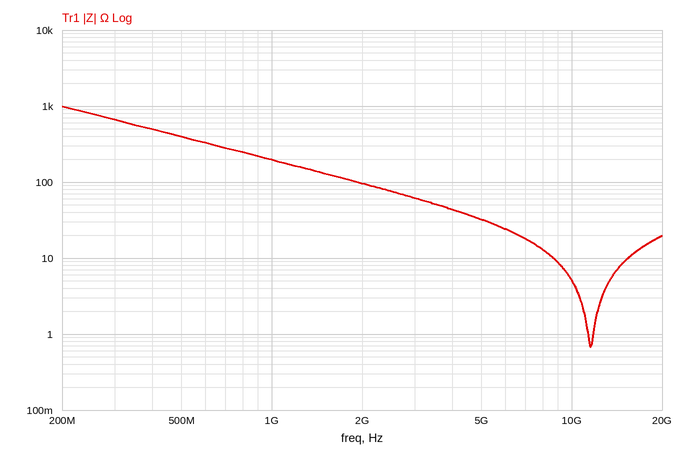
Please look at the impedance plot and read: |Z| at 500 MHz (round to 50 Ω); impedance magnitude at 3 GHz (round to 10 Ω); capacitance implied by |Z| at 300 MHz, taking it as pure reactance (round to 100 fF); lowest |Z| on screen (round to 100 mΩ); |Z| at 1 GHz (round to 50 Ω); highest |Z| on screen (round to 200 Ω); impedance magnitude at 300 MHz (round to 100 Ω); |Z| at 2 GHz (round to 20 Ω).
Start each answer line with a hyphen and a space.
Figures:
- 400 Ω
- 60 Ω
- 800 fF
- 700 mΩ
- 200 Ω
- 1.0 kΩ
- 700 Ω
- 100 Ω
